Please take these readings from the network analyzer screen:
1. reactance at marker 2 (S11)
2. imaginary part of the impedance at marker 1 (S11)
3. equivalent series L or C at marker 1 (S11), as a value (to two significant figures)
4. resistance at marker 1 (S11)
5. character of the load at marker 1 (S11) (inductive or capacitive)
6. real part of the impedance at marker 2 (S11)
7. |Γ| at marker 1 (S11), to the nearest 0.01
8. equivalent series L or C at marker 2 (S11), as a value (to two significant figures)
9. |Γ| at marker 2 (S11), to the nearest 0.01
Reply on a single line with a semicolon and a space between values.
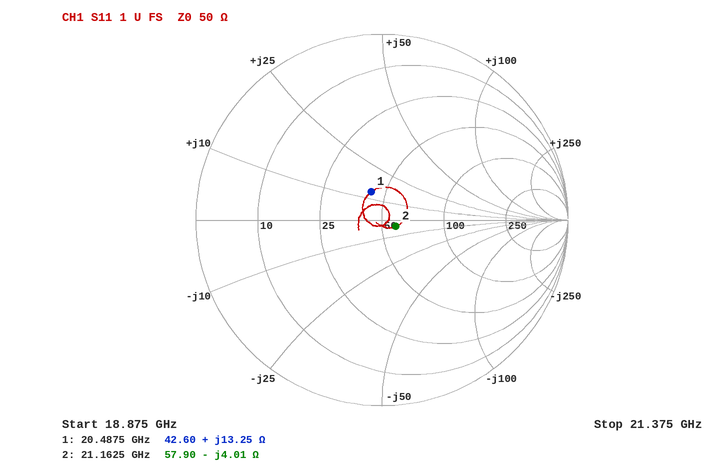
-4.01 Ω; +13.25 Ω; 100 pH; 42.60 Ω; inductive; 57.90 Ω; 0.16; 1.9 pF; 0.08
